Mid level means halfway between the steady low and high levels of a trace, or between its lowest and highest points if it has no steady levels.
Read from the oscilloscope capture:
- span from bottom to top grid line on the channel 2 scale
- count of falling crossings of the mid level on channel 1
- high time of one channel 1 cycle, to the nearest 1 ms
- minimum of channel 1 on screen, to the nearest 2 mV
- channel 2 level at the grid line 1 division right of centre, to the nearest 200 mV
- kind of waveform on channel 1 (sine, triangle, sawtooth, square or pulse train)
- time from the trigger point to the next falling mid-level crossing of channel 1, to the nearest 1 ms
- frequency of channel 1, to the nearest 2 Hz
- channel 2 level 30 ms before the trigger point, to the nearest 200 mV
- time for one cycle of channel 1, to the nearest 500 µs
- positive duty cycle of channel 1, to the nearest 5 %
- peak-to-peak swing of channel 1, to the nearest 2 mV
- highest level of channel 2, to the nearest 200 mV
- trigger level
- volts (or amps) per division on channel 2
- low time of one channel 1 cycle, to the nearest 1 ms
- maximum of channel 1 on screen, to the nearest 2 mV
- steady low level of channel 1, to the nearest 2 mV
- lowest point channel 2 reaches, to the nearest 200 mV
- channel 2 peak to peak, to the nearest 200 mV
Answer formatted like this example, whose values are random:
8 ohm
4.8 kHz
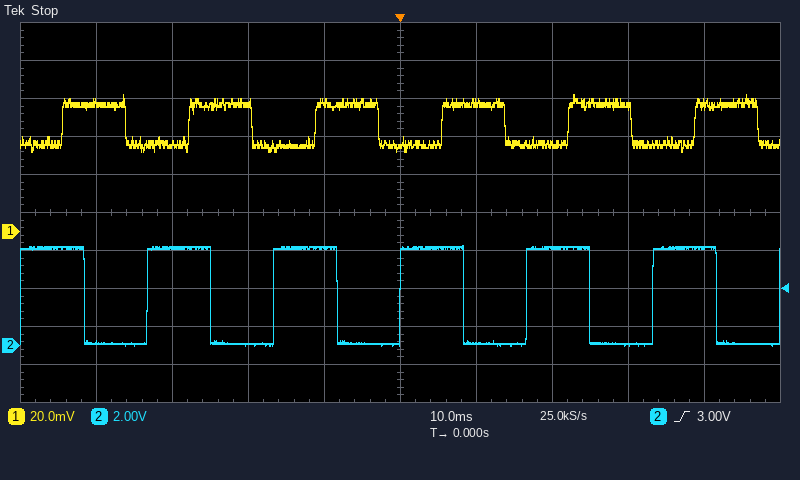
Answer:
20 V
6
8 ms
42 mV
200 mV
square
14 ms
60 Hz
5.2 V
16.5 ms
50 %
30 mV
5.2 V
3.00 V
2 V
8 ms
72 mV
46 mV
0.0 V
5.2 V
